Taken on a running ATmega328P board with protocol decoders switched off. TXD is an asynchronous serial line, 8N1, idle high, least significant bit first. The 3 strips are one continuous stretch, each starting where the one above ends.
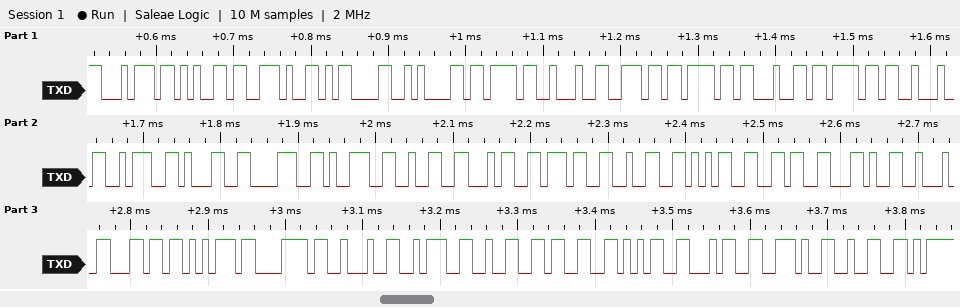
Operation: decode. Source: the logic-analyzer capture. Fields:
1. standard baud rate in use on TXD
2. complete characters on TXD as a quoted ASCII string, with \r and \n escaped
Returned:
115200 baud
"te.\r\n{\"nodo\":189247256,\"lux\":2354.2"
